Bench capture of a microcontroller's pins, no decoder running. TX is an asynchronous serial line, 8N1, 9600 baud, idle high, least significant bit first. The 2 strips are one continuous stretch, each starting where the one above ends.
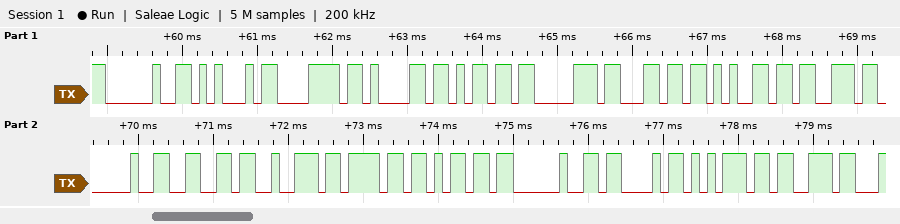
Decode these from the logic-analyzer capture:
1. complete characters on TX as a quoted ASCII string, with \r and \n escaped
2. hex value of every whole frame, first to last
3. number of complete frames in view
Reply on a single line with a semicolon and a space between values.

" Examples from Cus"; 0x20 0x45 0x78 0x61 0x6D 0x70 0x6C 0x65 0x73 0x20 0x66 0x72 0x6F 0x6D 0x20 0x43 0x75 0x73; 18
